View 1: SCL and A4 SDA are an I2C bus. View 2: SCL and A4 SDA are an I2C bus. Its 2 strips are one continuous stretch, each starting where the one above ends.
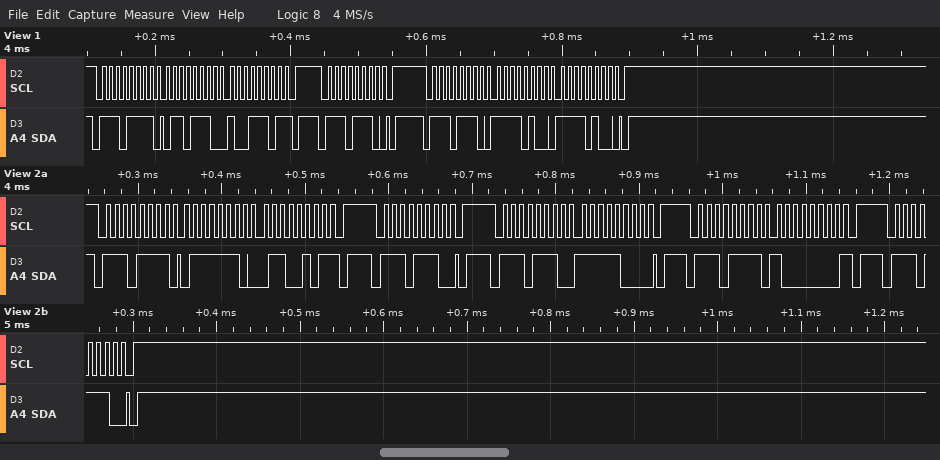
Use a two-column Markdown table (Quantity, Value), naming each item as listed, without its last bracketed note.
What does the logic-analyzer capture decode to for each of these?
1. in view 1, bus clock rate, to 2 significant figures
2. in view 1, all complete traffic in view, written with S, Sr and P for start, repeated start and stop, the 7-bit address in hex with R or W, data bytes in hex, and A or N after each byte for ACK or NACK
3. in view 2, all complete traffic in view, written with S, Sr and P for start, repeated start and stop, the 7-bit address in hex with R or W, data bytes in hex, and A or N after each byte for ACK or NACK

| Quantity | Value |
|---|---|
| in view 1, bus clock rate, to 2 significant figures | 100 kHz |
| in view 1, all complete traffic in view, written with S, Sr and P for start, repeated start and stop, the 7-bit address in hex with R or W, data bytes in hex, and A or N after each byte for ACK or NACK | S 77R A 6E A 9D N P S 77W A P S 77W A F4 A F4 A P |
| in view 2, all complete traffic in view, written with S, Sr and P for start, repeated start and stop, the 7-bit address in hex with R or W, data bytes in hex, and A or N after each byte for ACK or NACK | S 77R A 7E A 65 N P S 77W A P S 77W A F8 A P S 77R A 80 N P S 77W A P |
